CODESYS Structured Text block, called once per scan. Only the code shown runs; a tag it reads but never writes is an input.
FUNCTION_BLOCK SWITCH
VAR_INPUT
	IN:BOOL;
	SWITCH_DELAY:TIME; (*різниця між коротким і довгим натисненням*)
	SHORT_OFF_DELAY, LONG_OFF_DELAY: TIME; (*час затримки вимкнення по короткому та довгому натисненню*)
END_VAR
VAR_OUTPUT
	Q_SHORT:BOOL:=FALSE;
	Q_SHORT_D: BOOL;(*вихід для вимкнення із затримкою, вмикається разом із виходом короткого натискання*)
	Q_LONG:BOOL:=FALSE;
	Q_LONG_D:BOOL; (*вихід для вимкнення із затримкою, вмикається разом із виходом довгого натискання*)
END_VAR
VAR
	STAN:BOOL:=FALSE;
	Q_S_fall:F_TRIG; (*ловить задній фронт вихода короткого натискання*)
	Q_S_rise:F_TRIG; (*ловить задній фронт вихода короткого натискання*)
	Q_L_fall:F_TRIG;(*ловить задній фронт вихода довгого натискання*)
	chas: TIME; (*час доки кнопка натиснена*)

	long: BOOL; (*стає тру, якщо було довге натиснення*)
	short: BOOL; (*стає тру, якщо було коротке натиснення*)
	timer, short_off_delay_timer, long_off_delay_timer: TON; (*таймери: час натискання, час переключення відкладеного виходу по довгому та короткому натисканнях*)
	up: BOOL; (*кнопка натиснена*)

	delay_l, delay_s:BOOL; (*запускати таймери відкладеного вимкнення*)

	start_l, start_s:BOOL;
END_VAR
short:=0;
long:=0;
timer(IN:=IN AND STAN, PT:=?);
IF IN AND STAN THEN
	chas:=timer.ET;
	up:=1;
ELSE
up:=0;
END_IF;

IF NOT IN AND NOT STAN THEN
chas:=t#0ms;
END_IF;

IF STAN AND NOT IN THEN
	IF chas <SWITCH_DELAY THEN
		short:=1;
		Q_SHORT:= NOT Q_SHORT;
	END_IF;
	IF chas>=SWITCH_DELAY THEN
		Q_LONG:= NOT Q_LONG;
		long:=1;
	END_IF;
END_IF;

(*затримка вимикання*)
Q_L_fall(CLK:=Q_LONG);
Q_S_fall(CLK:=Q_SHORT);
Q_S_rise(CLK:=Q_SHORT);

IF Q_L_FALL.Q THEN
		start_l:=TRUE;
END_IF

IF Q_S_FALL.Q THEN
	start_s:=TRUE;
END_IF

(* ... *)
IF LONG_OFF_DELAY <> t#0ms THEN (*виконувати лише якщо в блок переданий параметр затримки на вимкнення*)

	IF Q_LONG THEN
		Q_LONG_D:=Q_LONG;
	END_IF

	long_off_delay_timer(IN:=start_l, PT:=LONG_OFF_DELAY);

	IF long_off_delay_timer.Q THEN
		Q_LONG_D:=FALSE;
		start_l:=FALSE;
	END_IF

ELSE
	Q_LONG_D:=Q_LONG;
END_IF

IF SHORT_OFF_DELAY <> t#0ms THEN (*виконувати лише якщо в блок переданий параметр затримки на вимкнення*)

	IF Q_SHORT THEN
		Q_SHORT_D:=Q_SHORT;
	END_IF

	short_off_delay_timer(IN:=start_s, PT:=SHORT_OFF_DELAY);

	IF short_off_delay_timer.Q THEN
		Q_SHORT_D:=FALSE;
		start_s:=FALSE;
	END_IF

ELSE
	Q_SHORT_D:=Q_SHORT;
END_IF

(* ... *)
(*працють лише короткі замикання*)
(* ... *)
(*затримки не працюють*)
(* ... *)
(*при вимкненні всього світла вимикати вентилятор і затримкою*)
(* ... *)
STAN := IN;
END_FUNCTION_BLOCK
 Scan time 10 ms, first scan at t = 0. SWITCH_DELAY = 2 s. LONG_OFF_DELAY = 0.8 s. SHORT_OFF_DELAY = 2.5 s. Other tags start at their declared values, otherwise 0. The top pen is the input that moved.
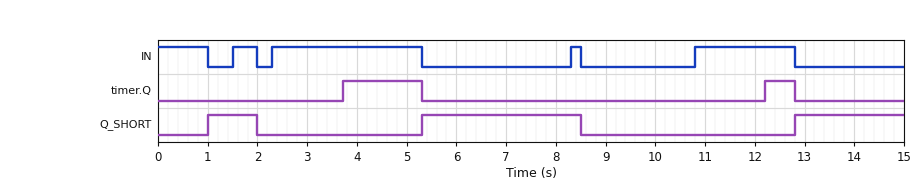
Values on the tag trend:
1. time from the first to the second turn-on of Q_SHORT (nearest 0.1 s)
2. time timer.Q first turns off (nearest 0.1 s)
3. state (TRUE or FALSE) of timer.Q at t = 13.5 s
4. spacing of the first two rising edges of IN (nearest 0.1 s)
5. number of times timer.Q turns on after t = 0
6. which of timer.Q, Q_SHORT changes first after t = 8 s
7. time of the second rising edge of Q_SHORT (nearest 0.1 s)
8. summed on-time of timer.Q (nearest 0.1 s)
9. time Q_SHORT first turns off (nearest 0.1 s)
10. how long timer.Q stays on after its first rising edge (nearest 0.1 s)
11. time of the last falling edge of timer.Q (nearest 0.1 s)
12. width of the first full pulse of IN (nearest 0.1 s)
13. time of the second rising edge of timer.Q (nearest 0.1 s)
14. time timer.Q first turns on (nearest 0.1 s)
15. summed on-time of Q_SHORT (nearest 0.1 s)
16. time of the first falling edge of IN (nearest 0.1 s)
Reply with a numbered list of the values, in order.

1. 4.3 s
2. 5.3 s
3. FALSE
4. 0.8 s
5. 2
6. Q_SHORT
7. 5.3 s
8. 2.2 s
9. 2.0 s
10. 1.6 s
11. 12.8 s
12. 0.5 s
13. 12.2 s
14. 3.7 s
15. 6.4 s
16. 1.0 s
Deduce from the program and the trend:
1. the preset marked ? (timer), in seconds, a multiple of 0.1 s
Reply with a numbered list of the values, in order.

1. 1.4 s
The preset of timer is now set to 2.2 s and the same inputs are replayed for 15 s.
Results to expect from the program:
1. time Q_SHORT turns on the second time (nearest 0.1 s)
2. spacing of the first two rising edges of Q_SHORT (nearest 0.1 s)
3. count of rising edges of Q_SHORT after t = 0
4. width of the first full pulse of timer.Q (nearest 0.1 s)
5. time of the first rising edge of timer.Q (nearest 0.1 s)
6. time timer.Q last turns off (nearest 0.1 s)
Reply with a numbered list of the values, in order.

1. 8.5 s
2. 7.5 s
3. 2
4. 0.8 s
5. 4.5 s
6. 5.3 s
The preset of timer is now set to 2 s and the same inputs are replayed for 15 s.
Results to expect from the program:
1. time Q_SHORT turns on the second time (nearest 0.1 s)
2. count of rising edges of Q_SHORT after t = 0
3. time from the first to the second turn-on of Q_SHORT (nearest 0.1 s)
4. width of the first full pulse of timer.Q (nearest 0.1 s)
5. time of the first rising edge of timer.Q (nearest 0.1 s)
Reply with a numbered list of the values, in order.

1. 8.5 s
2. 2
3. 7.5 s
4. 1.0 s
5. 4.3 s
